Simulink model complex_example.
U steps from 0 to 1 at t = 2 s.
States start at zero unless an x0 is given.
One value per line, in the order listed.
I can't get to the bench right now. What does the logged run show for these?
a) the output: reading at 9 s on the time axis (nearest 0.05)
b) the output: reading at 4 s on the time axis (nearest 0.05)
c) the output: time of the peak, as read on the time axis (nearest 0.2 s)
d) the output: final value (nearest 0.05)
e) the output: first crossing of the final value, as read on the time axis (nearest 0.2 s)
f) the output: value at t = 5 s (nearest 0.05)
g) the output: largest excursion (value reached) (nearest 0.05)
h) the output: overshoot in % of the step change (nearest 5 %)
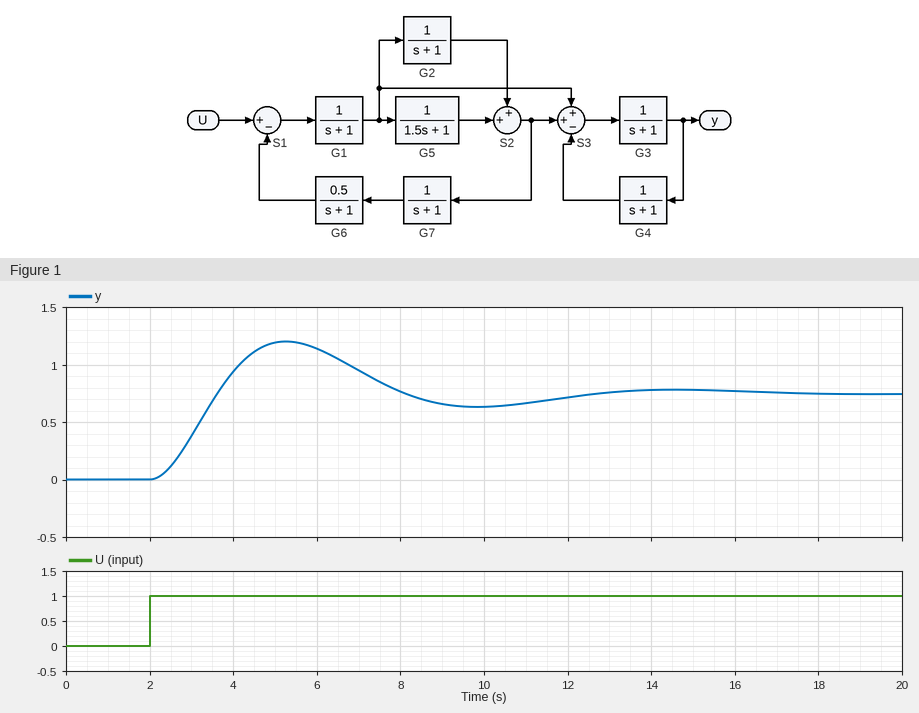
0.65
0.95
5.2 s
0.75
3.6 s
1.20
1.20
60 %
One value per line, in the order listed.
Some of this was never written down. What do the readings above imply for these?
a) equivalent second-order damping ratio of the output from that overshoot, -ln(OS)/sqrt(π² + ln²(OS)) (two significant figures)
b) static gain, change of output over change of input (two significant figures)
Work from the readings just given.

0.16
0.75
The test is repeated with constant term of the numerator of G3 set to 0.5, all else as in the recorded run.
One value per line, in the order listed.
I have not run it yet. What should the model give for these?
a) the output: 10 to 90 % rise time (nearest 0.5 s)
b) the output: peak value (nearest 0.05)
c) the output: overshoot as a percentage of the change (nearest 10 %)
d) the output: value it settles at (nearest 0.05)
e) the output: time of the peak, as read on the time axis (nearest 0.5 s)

1.5 s
0.75
50 %
0.50
5.5 s
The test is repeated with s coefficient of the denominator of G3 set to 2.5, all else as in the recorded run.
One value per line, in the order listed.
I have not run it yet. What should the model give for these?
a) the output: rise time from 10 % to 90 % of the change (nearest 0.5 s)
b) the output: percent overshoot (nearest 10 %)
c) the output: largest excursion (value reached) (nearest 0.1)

1.5 s
40 %
1.1
